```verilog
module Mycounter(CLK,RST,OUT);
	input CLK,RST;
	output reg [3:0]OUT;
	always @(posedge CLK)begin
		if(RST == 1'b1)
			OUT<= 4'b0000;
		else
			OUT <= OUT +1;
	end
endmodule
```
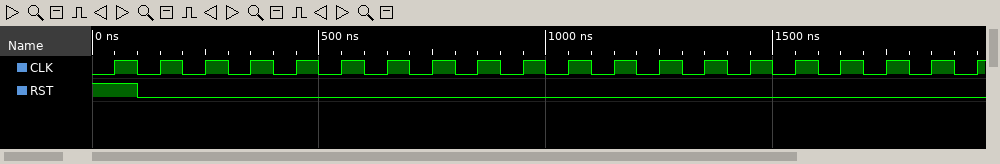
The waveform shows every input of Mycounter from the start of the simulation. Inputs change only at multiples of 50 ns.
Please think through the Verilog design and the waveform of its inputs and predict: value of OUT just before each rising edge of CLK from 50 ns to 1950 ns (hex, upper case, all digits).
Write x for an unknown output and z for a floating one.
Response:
x, 0, 1, 2, 3, 4, 5, 6, 7, 8, 9, A, B, C, D, E, F, 0, 1, 2
